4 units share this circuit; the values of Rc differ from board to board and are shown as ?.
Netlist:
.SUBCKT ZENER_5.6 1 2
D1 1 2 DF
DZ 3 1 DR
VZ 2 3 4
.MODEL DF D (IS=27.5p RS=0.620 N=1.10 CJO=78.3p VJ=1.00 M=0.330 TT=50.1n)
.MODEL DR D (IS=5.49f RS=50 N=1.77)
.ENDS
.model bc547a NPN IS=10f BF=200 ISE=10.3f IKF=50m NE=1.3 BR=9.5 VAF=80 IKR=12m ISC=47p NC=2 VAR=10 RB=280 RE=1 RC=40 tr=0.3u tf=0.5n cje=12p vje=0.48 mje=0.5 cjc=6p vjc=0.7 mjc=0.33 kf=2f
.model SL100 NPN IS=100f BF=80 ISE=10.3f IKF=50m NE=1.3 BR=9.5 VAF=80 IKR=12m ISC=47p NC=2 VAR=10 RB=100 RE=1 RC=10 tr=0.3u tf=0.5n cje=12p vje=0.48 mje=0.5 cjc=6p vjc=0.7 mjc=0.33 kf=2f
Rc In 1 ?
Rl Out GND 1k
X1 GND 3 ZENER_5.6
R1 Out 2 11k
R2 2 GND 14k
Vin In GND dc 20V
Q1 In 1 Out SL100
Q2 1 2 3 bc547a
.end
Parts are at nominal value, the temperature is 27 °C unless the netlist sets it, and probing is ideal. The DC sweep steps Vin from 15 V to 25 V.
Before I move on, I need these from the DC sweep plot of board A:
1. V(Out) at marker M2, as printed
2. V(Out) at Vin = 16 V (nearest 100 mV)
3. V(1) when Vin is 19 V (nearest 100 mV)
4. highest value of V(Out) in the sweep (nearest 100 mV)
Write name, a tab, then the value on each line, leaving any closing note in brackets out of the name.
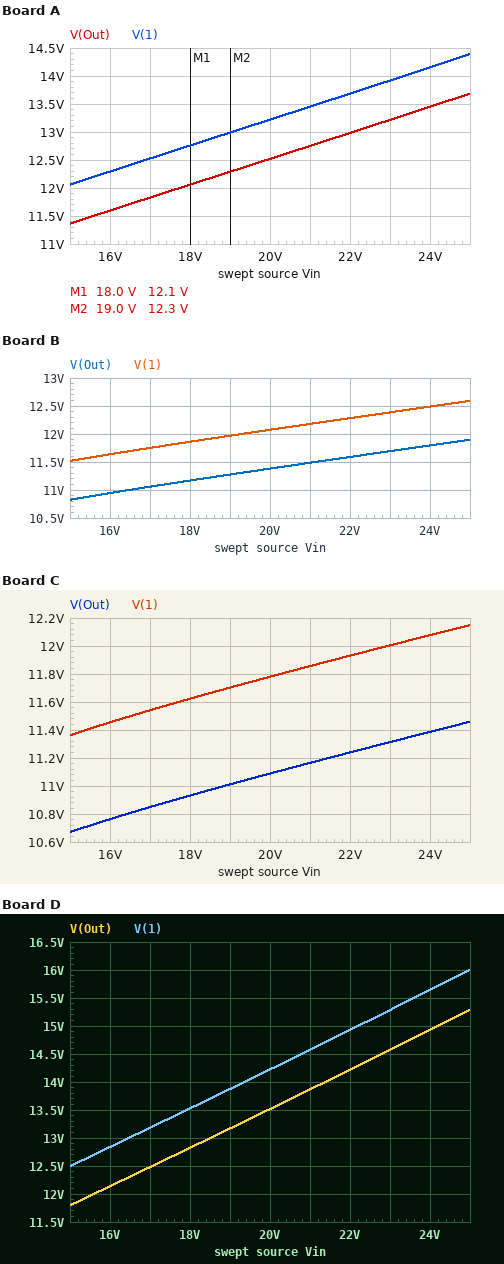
V(Out) at marker M2, as printed	12.3 V
V(Out) at Vin = 16 V	11.6 V
V(1) when Vin is 19 V	13.0 V
highest value of V(Out) in the sweep	13.7 V
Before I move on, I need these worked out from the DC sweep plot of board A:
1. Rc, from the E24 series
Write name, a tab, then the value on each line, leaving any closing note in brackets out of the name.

Rc, from the E24 series	680 Ω
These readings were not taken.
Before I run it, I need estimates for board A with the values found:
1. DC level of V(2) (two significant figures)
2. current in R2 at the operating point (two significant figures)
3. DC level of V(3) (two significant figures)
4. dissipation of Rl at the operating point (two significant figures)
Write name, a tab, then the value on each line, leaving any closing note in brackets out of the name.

DC level of V(2)	6.5 V
current in R2 at the operating point	470 µA
DC level of V(3)	5.8 V
dissipation of Rl at the operating point	160 mW
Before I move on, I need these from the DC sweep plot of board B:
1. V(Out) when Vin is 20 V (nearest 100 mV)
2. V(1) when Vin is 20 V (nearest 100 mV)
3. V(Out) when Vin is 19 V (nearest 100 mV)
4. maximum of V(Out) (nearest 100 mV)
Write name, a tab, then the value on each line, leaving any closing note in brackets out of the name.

V(Out) when Vin is 20 V	11.4 V
V(1) when Vin is 20 V	12.1 V
V(Out) when Vin is 19 V	11.3 V
maximum of V(Out)	11.9 V
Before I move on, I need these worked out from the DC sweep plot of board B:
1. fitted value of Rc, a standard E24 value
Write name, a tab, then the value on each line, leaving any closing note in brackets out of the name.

fitted value of Rc, a standard E24 value	1.8 kΩ
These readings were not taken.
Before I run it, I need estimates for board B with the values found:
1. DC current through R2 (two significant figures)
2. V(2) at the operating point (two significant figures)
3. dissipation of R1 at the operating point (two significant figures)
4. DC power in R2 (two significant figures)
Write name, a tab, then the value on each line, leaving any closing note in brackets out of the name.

DC current through R2	440 µA
V(2) at the operating point	6.2 V
dissipation of R1 at the operating point	2.5 mW
DC power in R2	2.7 mW
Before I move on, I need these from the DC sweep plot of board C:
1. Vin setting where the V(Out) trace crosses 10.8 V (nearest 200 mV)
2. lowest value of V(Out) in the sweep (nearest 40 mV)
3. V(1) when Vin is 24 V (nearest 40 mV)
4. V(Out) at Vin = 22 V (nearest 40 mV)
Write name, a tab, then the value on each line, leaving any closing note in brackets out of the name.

Vin setting where the V(Out) trace crosses 10.8 V	16.4 V
lowest value of V(Out) in the sweep	10.68 V
V(1) when Vin is 24 V	12.08 V
V(Out) at Vin = 22 V	11.24 V
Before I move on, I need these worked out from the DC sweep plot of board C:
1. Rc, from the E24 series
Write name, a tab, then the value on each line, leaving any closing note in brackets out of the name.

Rc, from the E24 series	2.7 kΩ
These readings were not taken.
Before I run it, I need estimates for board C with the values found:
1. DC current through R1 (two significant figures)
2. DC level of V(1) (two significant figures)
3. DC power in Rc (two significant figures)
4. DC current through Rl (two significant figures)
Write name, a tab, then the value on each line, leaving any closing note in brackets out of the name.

DC current through R1	460 µA
DC level of V(1)	12 V
DC power in Rc	25 mW
DC current through Rl	11 mA
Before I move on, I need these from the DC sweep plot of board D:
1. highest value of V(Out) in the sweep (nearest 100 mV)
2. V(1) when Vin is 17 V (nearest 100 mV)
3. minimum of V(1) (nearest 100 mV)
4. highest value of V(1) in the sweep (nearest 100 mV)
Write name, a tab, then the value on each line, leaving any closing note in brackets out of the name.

highest value of V(Out) in the sweep	15.3 V
V(1) when Vin is 17 V	13.2 V
minimum of V(1)	12.5 V
highest value of V(1) in the sweep	16.0 V
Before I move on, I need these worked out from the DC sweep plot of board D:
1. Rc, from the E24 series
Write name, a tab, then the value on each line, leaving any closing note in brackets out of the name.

Rc, from the E24 series	390 Ω
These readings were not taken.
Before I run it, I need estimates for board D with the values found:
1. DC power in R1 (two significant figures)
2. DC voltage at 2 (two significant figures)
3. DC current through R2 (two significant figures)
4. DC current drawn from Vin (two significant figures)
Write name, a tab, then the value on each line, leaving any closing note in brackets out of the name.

DC power in R1	4.1 mW
DC voltage at 2	6.8 V
DC current through R2	490 µA
DC current drawn from Vin	29 mA
